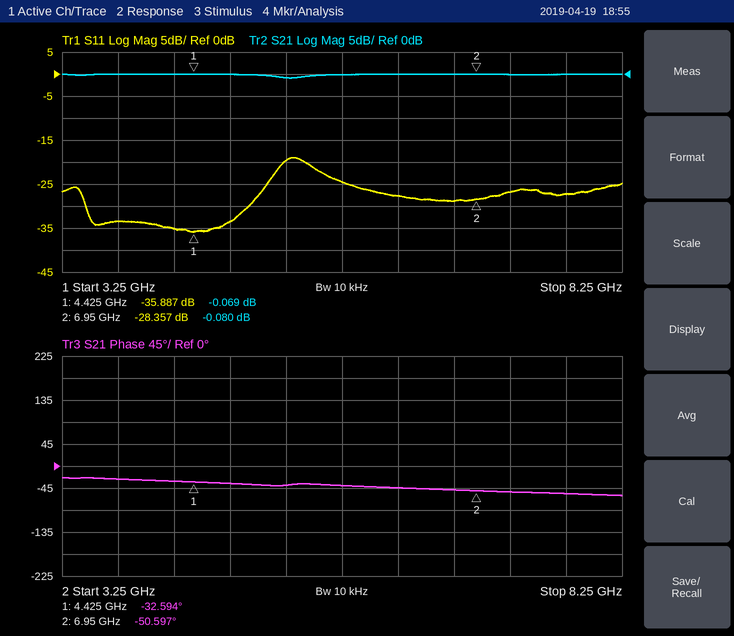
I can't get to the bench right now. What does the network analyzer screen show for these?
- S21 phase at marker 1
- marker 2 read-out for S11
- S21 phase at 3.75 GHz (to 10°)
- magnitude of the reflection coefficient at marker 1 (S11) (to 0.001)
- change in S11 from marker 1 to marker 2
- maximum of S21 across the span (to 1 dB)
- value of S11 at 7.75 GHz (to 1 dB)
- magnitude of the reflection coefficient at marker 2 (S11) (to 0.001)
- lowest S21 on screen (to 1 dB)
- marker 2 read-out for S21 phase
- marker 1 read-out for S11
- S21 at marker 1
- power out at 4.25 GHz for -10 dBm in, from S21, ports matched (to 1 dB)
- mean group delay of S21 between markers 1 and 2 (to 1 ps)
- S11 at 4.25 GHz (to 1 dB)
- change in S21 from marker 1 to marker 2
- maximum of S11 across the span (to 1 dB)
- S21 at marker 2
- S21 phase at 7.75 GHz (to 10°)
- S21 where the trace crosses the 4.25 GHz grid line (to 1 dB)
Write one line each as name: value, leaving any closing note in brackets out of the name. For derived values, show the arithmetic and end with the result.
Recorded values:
S21 phase at marker 1: -32.594°
marker 2 read-out for S11: -28.357 dB
S21 phase at 3.75 GHz: -30°
magnitude of the reflection coefficient at marker 1 (S11): 10^(-35.887/20) ≈ 0.016
change in S11 from marker 1 to marker 2: -28.357 − (-35.887) = 7.530 dB
maximum of S21 across the span: 0 dB
value of S11 at 7.75 GHz: -27 dB
magnitude of the reflection coefficient at marker 2 (S11): 10^(-28.357/20) ≈ 0.038
lowest S21 on screen: -1 dB
marker 2 read-out for S21 phase: -50.597°
marker 1 read-out for S11: -35.887 dB
S21 at marker 1: -0.069 dB
power out at 4.25 GHz for -10 dBm in, from S21, ports matched: -10 dBm + (0 dB) = -10 dBm
mean group delay of S21 between markers 1 and 2: −(-50.597° − (-32.594°))/(360° × 2.525 GHz) ≈ 20 ps
S11 at 4.25 GHz: -35 dB
change in S21 from marker 1 to marker 2: -0.08 − (-0.069) = -0.011 dB
maximum of S11 across the span: -19 dB
S21 at marker 2: -0.080 dB
S21 phase at 7.75 GHz: -60°
S21 where the trace crosses the 4.25 GHz grid line: 0 dB
